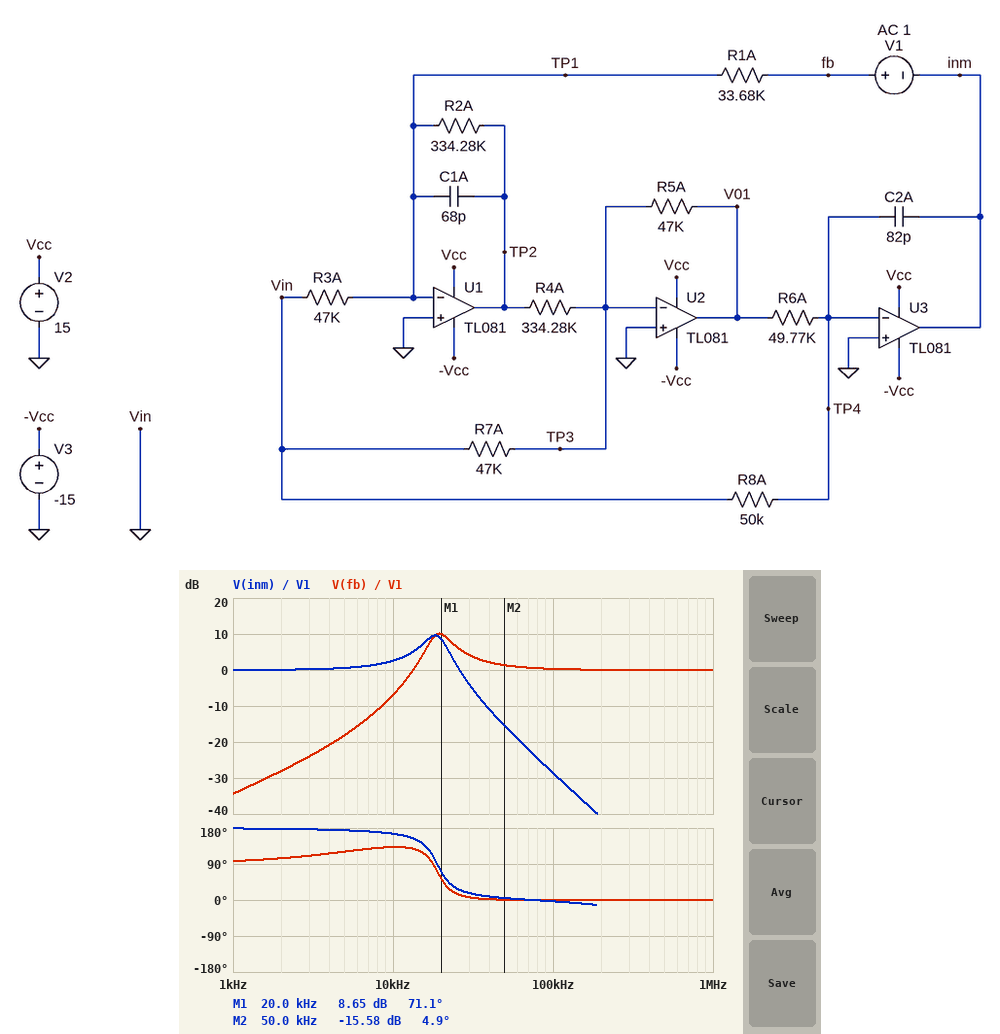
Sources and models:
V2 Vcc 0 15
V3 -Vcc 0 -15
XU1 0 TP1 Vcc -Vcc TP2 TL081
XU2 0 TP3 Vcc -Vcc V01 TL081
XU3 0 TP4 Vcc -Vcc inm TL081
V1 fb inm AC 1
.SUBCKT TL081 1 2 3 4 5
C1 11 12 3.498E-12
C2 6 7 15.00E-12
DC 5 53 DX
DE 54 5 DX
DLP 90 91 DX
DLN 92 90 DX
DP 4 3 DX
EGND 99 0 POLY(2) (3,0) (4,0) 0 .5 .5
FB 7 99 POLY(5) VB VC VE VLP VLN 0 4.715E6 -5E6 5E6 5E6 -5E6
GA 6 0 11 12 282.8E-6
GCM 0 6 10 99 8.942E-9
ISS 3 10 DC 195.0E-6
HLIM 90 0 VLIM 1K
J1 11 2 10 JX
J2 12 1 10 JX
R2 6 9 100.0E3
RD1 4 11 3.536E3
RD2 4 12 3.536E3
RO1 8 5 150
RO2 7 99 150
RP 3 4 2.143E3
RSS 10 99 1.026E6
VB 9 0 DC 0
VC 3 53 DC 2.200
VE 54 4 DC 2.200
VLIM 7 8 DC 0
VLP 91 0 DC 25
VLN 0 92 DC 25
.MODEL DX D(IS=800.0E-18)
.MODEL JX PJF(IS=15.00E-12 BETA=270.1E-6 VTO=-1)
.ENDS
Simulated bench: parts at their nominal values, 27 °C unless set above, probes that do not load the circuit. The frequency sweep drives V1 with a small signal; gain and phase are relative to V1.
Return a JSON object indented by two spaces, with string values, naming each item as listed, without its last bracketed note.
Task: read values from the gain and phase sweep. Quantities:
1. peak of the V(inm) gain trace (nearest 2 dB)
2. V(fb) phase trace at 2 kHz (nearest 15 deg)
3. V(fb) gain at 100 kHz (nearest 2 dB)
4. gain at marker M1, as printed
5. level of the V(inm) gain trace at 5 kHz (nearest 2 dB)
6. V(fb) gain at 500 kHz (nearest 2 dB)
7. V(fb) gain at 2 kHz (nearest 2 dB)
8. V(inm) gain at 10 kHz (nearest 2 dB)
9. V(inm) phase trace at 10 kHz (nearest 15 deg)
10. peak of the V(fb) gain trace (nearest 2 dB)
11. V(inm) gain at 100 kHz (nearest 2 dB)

{
  "peak of the V(inm) gain trace": "10 dB",
  "V(fb) phase trace at 2 kHz": "105 deg",
  "V(fb) gain at 100 kHz": "0 dB",
  "gain at marker M1, as printed": "8.65 dB",
  "level of the V(inm) gain trace at 5 kHz": "0 dB",
  "V(fb) gain at 500 kHz": "0 dB",
  "V(fb) gain at 2 kHz": "-28 dB",
  "V(inm) gain at 10 kHz": "2 dB",
  "V(inm) phase trace at 10 kHz": "165 deg",
  "peak of the V(fb) gain trace": "10 dB",
  "V(inm) gain at 100 kHz": "-28 dB"
}
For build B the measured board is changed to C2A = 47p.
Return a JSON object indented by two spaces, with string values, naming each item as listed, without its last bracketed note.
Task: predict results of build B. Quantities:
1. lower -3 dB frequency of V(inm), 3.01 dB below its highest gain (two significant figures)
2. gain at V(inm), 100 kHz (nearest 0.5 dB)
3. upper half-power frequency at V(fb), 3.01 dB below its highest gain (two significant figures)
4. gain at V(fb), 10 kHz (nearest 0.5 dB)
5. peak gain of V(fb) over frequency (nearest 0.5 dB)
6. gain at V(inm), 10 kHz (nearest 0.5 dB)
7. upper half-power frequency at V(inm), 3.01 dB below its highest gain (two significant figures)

{
  "lower -3 dB frequency of V(inm), 3.01 dB below its highest gain": "21 kHz",
  "gain at V(inm), 100 kHz": "-23.5 dB",
  "upper half-power frequency at V(fb), 3.01 dB below its highest gain": "29 kHz",
  "gain at V(fb), 10 kHz": "-12.5 dB",
  "peak gain of V(fb) over frequency": "12.5 dB",
  "gain at V(inm), 10 kHz": "1.5 dB",
  "upper half-power frequency at V(inm), 3.01 dB below its highest gain": "27 kHz"
}
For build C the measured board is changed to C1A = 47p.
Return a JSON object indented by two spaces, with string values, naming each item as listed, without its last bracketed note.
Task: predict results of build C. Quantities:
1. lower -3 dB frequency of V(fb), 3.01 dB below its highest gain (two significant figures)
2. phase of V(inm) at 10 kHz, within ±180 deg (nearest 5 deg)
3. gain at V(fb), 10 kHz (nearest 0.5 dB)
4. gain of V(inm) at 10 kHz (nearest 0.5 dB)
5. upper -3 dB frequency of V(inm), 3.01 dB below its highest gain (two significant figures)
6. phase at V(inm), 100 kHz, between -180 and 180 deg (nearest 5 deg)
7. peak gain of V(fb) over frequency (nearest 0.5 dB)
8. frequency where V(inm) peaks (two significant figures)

{
  "lower -3 dB frequency of V(fb), 3.01 dB below its highest gain": "20 kHz",
  "phase of V(inm) at 10 kHz, within ±180 deg": "165 deg",
  "gain at V(fb), 10 kHz": "-9.5 dB",
  "gain of V(inm) at 10 kHz": "1.5 dB",
  "upper -3 dB frequency of V(inm), 3.01 dB below its highest gain": "26 kHz",
  "phase at V(inm), 100 kHz, between -180 and 180 deg": "0 deg",
  "peak gain of V(fb) over frequency": "9.0 dB",
  "frequency where V(inm) peaks": "22 kHz"
}
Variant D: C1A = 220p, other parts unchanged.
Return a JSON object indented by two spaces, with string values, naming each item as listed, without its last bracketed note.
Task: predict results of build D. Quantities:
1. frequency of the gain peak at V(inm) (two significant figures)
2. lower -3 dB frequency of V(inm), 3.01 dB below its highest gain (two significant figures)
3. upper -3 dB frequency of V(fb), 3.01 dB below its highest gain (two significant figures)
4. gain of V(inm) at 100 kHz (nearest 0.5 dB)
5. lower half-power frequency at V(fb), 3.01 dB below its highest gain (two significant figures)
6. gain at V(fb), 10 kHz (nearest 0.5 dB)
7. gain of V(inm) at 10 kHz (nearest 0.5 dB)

{
  "frequency of the gain peak at V(inm)": "11 kHz",
  "lower -3 dB frequency of V(inm), 3.01 dB below its highest gain": "9.5 kHz",
  "upper -3 dB frequency of V(fb), 3.01 dB below its highest gain": "12 kHz",
  "gain of V(inm) at 100 kHz": "-39.0 dB",
  "lower half-power frequency at V(fb), 3.01 dB below its highest gain": "9.9 kHz",
  "gain at V(fb), 10 kHz": "12.5 dB",
  "gain of V(inm) at 10 kHz": "13.5 dB"
}
